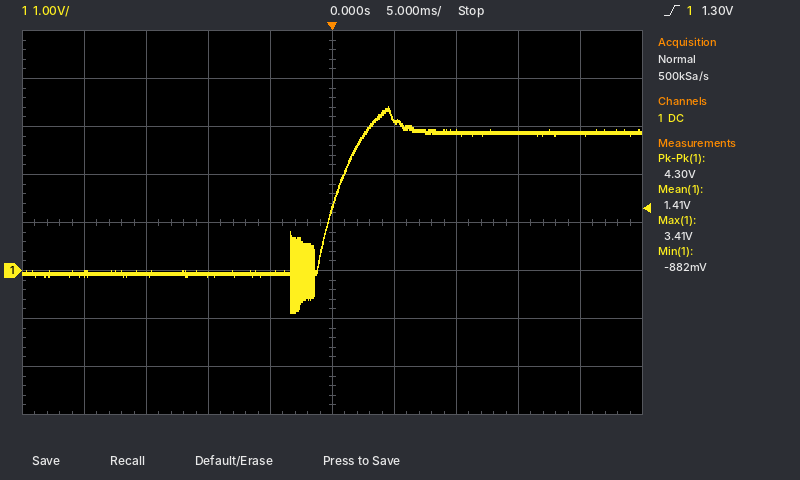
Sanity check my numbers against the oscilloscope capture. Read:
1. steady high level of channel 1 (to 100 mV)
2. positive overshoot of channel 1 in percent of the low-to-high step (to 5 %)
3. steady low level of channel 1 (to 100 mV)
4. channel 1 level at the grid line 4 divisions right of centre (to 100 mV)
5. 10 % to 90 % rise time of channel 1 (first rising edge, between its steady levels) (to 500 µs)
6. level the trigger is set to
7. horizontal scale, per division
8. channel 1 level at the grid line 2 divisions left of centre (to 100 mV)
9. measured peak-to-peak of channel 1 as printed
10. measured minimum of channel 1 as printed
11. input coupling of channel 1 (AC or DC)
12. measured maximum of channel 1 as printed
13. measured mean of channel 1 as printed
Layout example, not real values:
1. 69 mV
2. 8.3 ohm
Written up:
1. 2.9 V
2. 20 %
3. -100 mV
4. 2.9 V
5. 3.0 ms
6. 1.30 V
7. 5 ms
8. -100 mV
9. 4.30 V
10. -882 mV
11. DC
12. 3.41 V
13. 1.41 V
